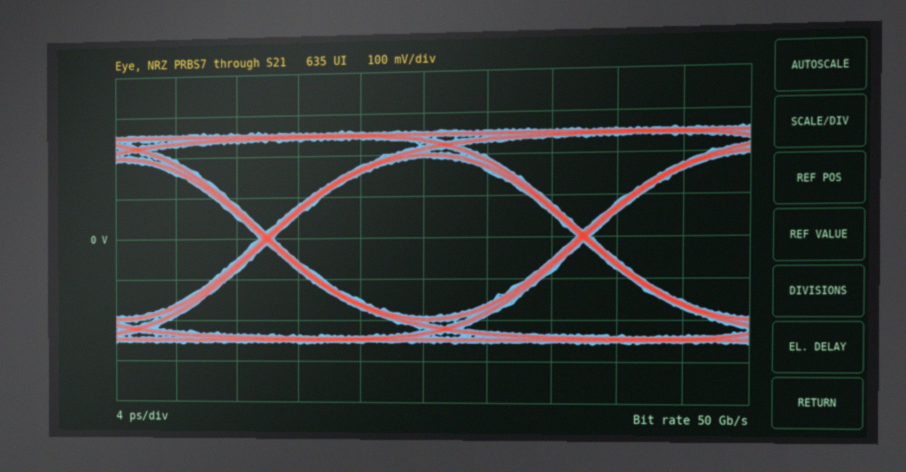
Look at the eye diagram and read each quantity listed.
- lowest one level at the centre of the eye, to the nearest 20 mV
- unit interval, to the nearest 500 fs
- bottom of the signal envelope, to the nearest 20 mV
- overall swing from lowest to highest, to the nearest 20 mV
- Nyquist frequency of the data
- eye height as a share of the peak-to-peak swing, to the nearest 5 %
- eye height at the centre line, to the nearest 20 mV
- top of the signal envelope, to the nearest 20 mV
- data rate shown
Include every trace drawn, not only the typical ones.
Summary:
200 mV
20.0 ps
-260 mV
520 mV
25 GHz
75 %
380 mV
260 mV
50 Gb/s
